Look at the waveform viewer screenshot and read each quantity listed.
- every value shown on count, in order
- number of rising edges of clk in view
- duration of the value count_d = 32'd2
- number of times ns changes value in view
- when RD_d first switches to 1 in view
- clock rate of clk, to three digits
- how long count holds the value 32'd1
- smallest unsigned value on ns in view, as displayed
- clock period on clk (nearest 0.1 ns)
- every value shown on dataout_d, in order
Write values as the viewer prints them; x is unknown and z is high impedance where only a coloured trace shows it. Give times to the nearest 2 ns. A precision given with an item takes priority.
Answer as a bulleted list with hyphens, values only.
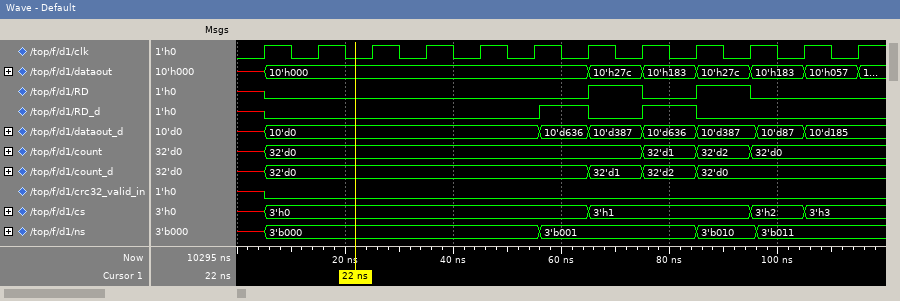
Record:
- x, 32'd0, 32'd1, 32'd2, 32'd0
- 12
- 10 ns
- 4
- 56 ns
- 100 MHz
- 10 ns
- 3'b000
- 10 ns
- x, 10'd0, 10'd636, 10'd387, 10'd636, 10'd387, 10'd87, 10'd185
